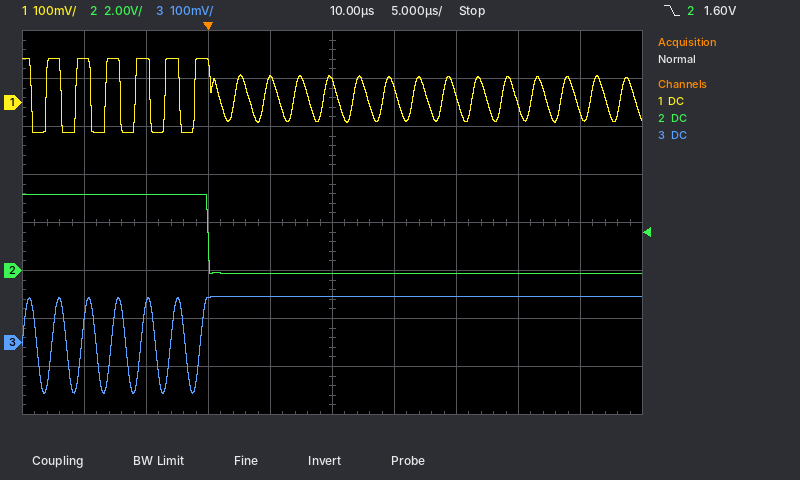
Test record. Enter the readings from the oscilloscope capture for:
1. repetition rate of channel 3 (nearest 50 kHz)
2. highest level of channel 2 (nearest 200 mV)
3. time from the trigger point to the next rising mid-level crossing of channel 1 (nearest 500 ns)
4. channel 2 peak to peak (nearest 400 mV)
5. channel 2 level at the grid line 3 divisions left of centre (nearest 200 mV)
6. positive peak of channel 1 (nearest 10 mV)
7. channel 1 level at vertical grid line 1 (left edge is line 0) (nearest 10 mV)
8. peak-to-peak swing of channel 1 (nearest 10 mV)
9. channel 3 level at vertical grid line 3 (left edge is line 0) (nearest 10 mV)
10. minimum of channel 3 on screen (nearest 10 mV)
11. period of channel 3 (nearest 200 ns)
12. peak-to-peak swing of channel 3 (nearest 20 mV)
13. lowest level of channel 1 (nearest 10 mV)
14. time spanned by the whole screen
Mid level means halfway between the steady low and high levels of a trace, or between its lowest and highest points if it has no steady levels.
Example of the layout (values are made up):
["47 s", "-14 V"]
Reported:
["400 kHz", "3.2 V", "2.0 µs", "3.2 V", "3.2 V", "90 mV", "90 mV", "150 mV", "90 mV", "-110 mV", "2.4 µs", "200 mV", "-60 mV", "50 µs"]
